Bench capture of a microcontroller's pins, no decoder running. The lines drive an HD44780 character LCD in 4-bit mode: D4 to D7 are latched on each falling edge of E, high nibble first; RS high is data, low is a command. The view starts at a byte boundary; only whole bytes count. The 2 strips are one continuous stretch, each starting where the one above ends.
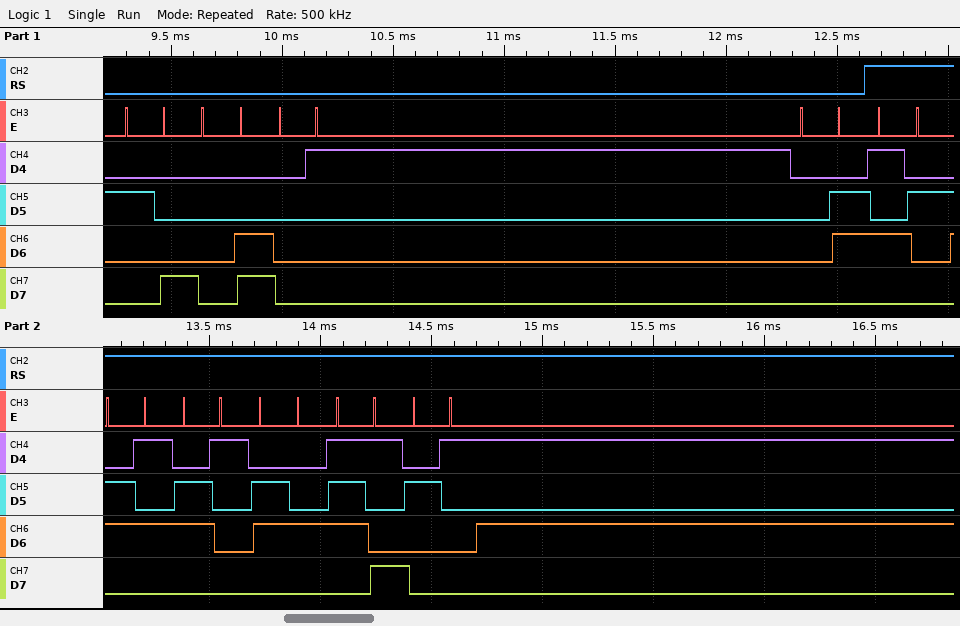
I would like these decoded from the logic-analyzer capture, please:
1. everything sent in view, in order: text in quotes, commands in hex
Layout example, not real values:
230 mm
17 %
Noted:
0x28 0x0C 0x01 0x06 "Ready!"
